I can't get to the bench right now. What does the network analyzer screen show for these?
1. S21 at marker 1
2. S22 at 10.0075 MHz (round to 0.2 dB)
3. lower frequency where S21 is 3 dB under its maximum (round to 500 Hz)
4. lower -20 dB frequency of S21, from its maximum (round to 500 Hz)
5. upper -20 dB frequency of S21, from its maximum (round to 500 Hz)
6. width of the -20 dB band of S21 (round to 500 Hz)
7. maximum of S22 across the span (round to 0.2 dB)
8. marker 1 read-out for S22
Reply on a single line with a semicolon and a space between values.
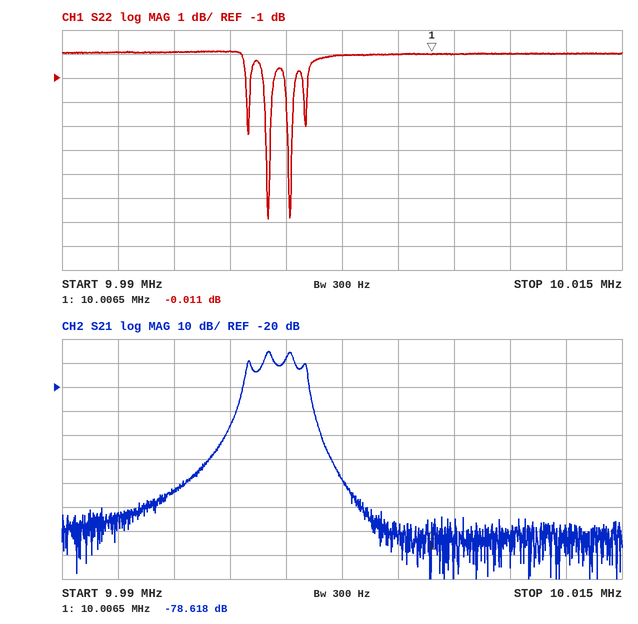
-78.618 dB; 0.0 dB; 9.9990 MHz; 9.9980 MHz; 10.0010 MHz; 3.0 kHz; 0.2 dB; -0.011 dB
